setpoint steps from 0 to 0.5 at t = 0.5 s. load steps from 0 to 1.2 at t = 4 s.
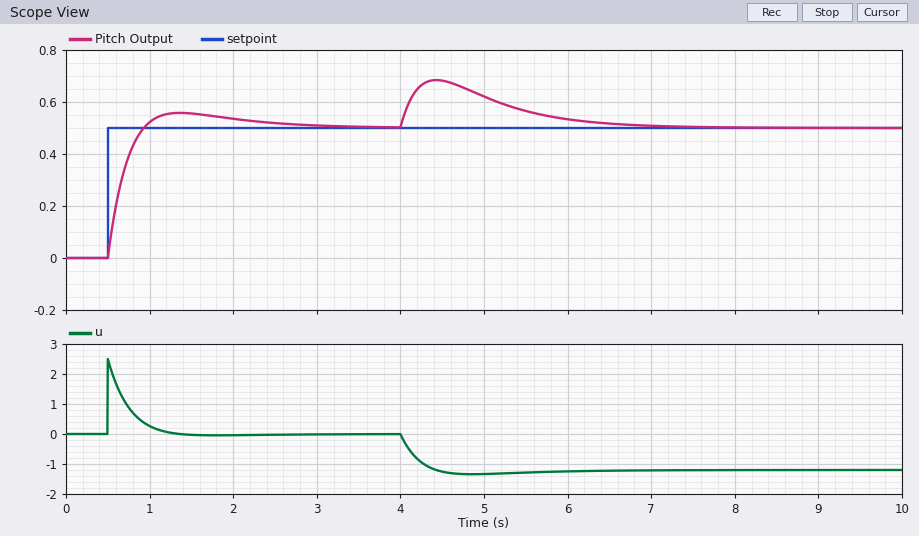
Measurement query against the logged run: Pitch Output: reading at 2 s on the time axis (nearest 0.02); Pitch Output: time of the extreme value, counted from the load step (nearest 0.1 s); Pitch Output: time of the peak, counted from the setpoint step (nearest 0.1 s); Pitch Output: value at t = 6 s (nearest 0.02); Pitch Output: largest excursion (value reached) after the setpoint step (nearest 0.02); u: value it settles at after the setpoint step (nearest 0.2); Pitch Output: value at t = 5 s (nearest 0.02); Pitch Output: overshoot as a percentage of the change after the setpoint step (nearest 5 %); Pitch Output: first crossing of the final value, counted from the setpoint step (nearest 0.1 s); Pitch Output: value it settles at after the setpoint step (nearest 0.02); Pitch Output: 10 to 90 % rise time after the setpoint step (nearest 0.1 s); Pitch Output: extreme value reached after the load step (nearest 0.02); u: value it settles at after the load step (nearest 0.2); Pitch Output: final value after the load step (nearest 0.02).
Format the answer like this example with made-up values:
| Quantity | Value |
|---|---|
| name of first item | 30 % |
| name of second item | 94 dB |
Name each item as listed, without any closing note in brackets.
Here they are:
| Quantity | Value |
|---|---|
| Pitch Output: reading at 2 s on the time axis | 0.54 |
| Pitch Output: time of the extreme value, counted from the load step | 0.4 s |
| Pitch Output: time of the peak, counted from the setpoint step | 0.9 s |
| Pitch Output: value at t = 6 s | 0.54 |
| Pitch Output: largest excursion (value reached) after the setpoint step | 0.56 |
| u: value it settles at after the setpoint step | 0.0 |
| Pitch Output: value at t = 5 s | 0.62 |
| Pitch Output: overshoot as a percentage of the change after the setpoint step | 10 % |
| Pitch Output: first crossing of the final value, counted from the setpoint step | 0.4 s |
| Pitch Output: value it settles at after the setpoint step | 0.50 |
| Pitch Output: 10 to 90 % rise time after the setpoint step | 0.3 s |
| Pitch Output: extreme value reached after the load step | 0.68 |
| u: value it settles at after the load step | -1.2 |
| Pitch Output: final value after the load step | 0.50 |
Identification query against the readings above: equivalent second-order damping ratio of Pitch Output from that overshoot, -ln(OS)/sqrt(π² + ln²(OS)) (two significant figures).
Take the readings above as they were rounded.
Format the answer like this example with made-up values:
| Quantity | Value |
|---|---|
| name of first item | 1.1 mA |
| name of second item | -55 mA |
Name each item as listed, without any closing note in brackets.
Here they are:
| Quantity | Value |
|---|---|
| equivalent second-order damping ratio of Pitch Output from that overshoot, -ln(OS)/sqrt(π² + ln²(OS)) | 0.59 |
